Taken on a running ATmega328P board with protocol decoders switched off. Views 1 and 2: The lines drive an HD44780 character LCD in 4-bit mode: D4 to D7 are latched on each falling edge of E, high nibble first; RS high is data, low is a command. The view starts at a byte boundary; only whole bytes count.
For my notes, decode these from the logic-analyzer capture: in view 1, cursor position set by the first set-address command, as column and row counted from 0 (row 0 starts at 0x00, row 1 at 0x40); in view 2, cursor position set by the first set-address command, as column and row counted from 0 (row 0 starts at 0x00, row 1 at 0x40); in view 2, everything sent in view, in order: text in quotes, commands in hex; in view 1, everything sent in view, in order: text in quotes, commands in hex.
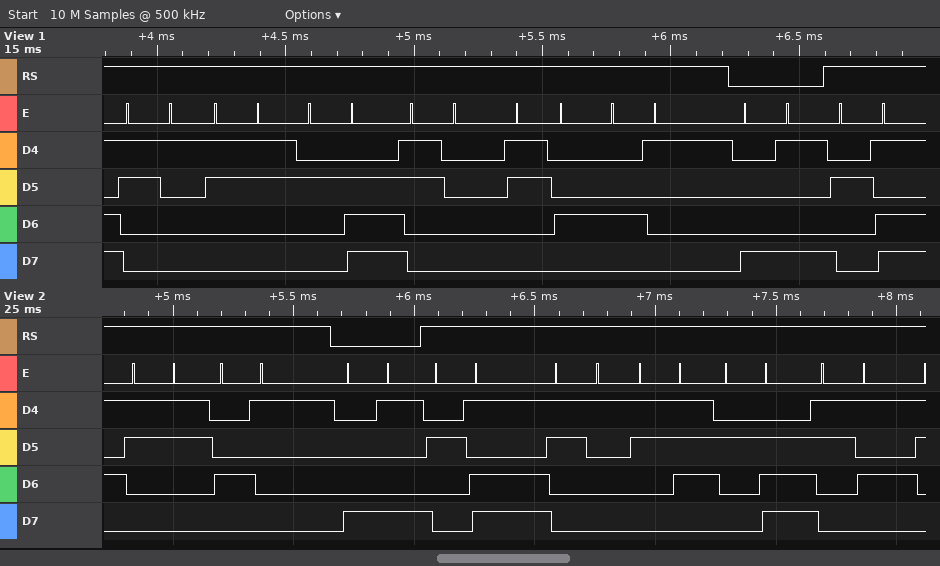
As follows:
column 9, row 0
column 9, row 0
"3A" 0x89 "-17.5"
"13.04A" 0x89 "-"
